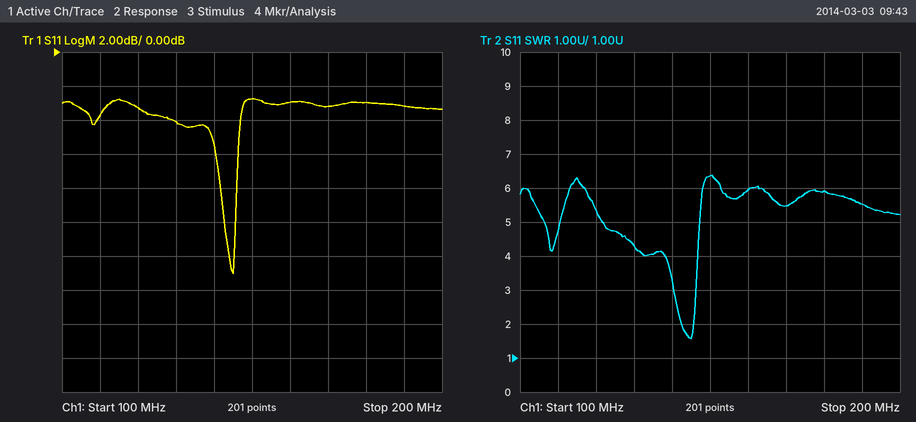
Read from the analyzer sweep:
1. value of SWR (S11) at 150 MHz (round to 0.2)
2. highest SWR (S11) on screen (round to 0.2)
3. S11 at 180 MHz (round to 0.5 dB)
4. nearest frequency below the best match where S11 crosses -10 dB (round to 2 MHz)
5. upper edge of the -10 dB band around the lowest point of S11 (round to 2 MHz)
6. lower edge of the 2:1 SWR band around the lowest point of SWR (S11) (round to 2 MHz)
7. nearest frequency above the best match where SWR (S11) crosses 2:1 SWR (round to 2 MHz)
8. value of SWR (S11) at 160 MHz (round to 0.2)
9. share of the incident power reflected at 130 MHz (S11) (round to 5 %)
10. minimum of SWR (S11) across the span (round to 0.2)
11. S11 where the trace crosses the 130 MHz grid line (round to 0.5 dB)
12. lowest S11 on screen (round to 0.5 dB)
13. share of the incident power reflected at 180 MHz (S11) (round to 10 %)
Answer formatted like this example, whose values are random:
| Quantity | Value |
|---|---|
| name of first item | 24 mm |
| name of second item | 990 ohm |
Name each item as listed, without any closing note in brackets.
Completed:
| Quantity | Value |
|---|---|
| value of SWR (S11) at 150 MHz | 6.4 |
| highest SWR (S11) on screen | 6.4 |
| S11 at 180 MHz | -3.0 dB |
| nearest frequency below the best match where S11 crosses -10 dB | 142 MHz |
| upper edge of the -10 dB band around the lowest point of S11 | 146 MHz |
| lower edge of the 2:1 SWR band around the lowest point of SWR (S11) | 142 MHz |
| nearest frequency above the best match where SWR (S11) crosses 2:1 SWR | 146 MHz |
| value of SWR (S11) at 160 MHz | 6.0 |
| share of the incident power reflected at 130 MHz (S11) | 40 % |
| minimum of SWR (S11) across the span | 1.6 |
| S11 where the trace crosses the 130 MHz grid line | -4.0 dB |
| lowest S11 on screen | -13.0 dB |
| share of the incident power reflected at 180 MHz (S11) | 50 % |
